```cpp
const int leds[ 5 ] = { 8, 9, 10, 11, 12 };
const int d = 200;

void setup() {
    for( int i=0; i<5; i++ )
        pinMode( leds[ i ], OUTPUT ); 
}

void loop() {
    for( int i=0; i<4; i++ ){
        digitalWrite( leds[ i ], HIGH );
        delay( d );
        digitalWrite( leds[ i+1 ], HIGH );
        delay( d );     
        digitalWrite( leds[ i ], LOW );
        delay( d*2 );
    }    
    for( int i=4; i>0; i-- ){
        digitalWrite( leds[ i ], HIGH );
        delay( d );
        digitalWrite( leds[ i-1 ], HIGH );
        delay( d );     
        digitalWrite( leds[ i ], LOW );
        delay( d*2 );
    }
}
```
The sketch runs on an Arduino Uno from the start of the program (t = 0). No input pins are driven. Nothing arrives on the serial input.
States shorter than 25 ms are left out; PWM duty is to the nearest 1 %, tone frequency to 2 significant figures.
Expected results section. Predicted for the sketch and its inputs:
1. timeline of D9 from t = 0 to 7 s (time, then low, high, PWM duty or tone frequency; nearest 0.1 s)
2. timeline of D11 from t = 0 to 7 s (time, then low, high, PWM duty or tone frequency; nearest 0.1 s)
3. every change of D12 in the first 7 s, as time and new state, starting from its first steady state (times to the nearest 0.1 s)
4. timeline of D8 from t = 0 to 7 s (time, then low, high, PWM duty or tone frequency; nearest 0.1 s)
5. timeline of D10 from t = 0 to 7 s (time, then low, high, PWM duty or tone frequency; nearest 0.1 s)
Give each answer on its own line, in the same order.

0 s low; 0.2 s high; 1.2 s low; 5 s high; 6 s low; 6.6 s high
0 s low; 1.8 s high; 2.8 s low; 3.4 s high; 4.4 s low
0 s low; 2.6 s high; 3.6 s low
0 s high; 0.4 s low; 5.8 s high; 6.8 s low
0 s low; 1 s high; 2 s low; 4.2 s high; 5.2 s low
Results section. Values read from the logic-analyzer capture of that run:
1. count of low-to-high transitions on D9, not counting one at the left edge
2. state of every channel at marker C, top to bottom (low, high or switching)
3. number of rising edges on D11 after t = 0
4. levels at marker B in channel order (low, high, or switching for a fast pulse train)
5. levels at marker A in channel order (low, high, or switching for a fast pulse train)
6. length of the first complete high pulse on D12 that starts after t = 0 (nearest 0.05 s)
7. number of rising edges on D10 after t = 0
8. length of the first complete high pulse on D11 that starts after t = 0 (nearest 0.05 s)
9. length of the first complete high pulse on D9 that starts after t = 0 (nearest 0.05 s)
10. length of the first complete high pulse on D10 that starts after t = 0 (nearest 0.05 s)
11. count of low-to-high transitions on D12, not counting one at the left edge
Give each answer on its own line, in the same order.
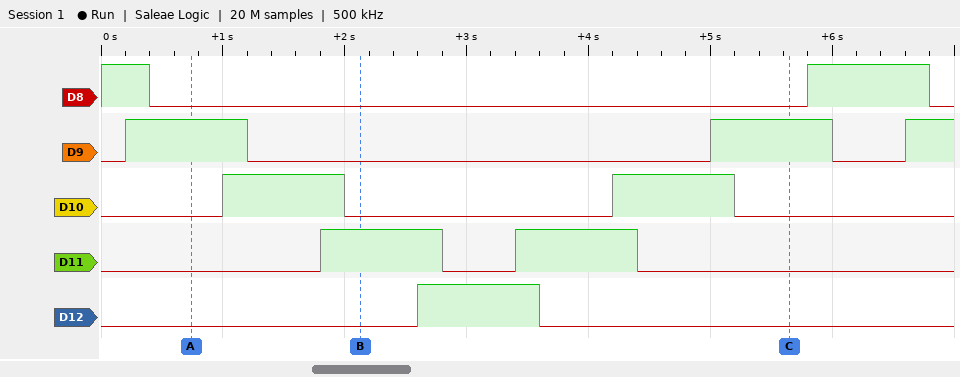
3
D8 low, D9 high, D10 low, D11 low, D12 low
2
D8 low, D9 low, D10 low, D11 high, D12 low
D8 low, D9 high, D10 low, D11 low, D12 low
1.00 s
2
1.00 s
1.00 s
1.00 s
1
